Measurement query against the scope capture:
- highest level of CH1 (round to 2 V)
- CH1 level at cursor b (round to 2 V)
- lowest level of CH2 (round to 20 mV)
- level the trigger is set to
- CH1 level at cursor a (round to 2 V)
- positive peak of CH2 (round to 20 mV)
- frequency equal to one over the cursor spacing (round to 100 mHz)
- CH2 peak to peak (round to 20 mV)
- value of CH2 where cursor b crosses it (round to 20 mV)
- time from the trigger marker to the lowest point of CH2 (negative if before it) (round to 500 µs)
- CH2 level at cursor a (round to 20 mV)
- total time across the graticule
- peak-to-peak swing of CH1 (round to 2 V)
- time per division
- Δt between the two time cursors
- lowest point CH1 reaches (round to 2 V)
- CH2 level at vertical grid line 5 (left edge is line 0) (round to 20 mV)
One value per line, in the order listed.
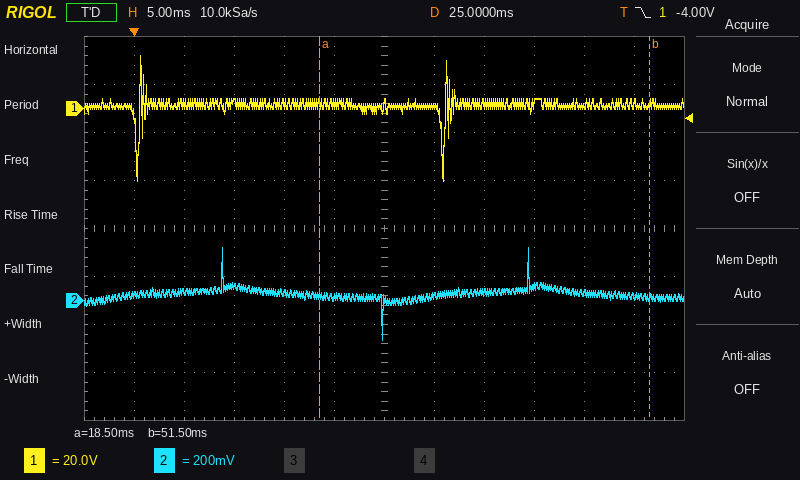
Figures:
22 V
2 V
-160 mV
-4.00 V
2 V
220 mV
30.3 Hz
380 mV
20 mV
+25.0 ms
20 mV
60 ms
52 V
5 ms
33.0 ms
-30 V
20 mV
